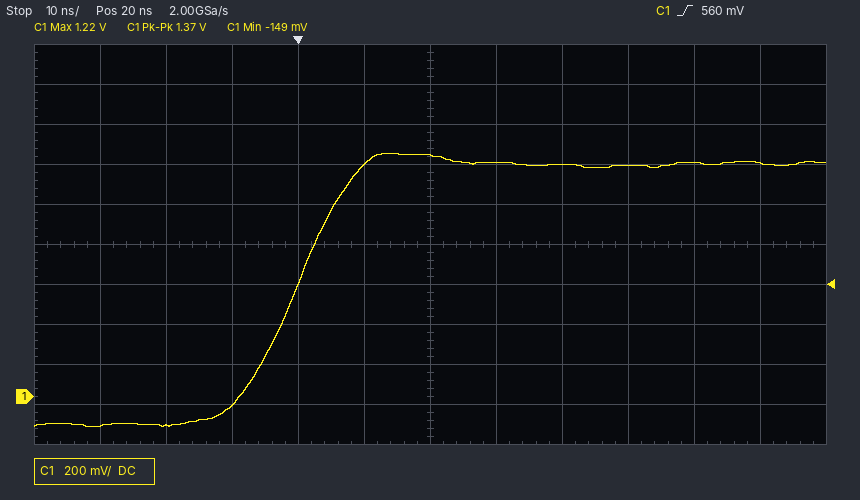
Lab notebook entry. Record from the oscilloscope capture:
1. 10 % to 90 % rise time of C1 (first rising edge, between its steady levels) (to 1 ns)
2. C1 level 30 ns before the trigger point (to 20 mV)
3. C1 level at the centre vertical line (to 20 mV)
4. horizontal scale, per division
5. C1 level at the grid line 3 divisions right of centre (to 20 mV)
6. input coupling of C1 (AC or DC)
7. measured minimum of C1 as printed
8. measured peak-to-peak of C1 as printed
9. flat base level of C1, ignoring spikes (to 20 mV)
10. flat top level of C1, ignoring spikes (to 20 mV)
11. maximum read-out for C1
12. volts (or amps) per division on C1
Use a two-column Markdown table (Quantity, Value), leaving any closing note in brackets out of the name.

| Quantity | Value |
|---|---|
| 10 % to 90 % rise time of C1 (first rising edge, between its steady levels) | 16 ns |
| C1 level 30 ns before the trigger point | -140 mV |
| C1 level at the centre vertical line | 1.20 V |
| horizontal scale, per division | 10 ns |
| C1 level at the grid line 3 divisions right of centre | 1.16 V |
| input coupling of C1 | DC |
| measured minimum of C1 as printed | -149 mV |
| measured peak-to-peak of C1 as printed | 1.37 V |
| flat base level of C1, ignoring spikes | -140 mV |
| flat top level of C1, ignoring spikes | 1.16 V |
| maximum read-out for C1 | 1.22 V |
| volts (or amps) per division on C1 | 200 mV |
